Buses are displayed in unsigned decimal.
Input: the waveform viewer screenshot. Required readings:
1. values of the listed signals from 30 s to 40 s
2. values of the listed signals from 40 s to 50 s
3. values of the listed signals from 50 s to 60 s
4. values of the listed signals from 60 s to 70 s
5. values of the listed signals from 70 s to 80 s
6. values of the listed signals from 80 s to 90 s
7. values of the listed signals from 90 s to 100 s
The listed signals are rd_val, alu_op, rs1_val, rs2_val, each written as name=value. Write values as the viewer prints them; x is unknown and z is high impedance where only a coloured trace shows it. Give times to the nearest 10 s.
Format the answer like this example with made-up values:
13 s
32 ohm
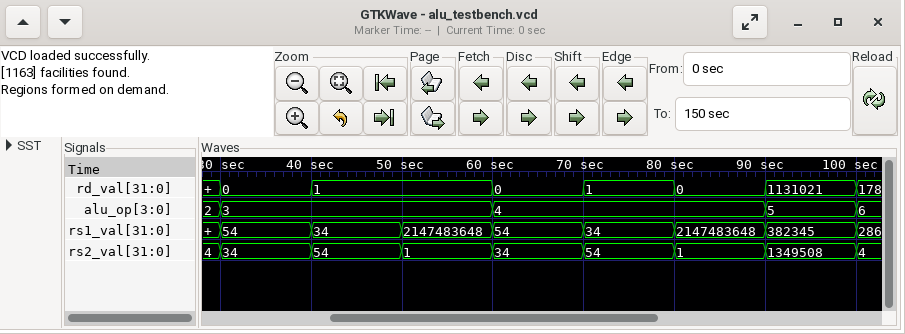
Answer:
rd_val=0, alu_op=3, rs1_val=54, rs2_val=34
rd_val=1, alu_op=3, rs1_val=34, rs2_val=54
rd_val=1, alu_op=3, rs1_val=2147483648, rs2_val=1
rd_val=0, alu_op=4, rs1_val=54, rs2_val=34
rd_val=1, alu_op=4, rs1_val=34, rs2_val=54
rd_val=0, alu_op=4, rs1_val=2147483648, rs2_val=1
rd_val=1131021, alu_op=5, rs1_val=382345, rs2_val=1349508
